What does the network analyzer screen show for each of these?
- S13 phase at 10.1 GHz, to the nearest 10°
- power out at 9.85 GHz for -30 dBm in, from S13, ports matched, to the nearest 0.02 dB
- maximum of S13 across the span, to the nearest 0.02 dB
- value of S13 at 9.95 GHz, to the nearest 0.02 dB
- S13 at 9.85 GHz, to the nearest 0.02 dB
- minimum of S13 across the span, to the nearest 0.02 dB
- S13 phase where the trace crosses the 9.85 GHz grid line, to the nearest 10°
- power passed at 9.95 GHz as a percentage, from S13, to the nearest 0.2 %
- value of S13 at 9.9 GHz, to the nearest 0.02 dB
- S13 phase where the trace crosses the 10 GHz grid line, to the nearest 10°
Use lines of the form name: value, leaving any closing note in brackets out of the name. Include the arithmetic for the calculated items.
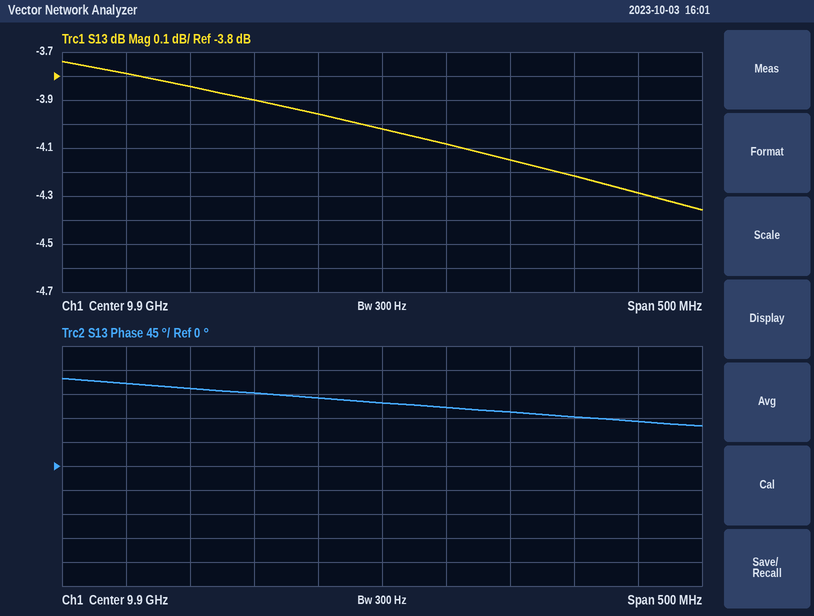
S13 phase at 10.1 GHz, to the nearest 10°: 80°
power out at 9.85 GHz for -30 dBm in, from S13, ports matched, to the nearest 0.02 dB: -30 dBm + (-3.96 dB) = -33.96 dBm
maximum of S13 across the span, to the nearest 0.02 dB: -3.74 dB
value of S13 at 9.95 GHz, to the nearest 0.02 dB: -4.08 dB
S13 at 9.85 GHz, to the nearest 0.02 dB: -3.96 dB
minimum of S13 across the span, to the nearest 0.02 dB: -4.36 dB
S13 phase where the trace crosses the 9.85 GHz grid line, to the nearest 10°: 130°
power passed at 9.95 GHz as a percentage, from S13, to the nearest 0.2 %: 10^(-4.08/10) ≈ 39.1 %, so 39.0 % to the nearest 0.2 %
value of S13 at 9.9 GHz, to the nearest 0.02 dB: -4.02 dB
S13 phase where the trace crosses the 10 GHz grid line, to the nearest 10°: 100°
